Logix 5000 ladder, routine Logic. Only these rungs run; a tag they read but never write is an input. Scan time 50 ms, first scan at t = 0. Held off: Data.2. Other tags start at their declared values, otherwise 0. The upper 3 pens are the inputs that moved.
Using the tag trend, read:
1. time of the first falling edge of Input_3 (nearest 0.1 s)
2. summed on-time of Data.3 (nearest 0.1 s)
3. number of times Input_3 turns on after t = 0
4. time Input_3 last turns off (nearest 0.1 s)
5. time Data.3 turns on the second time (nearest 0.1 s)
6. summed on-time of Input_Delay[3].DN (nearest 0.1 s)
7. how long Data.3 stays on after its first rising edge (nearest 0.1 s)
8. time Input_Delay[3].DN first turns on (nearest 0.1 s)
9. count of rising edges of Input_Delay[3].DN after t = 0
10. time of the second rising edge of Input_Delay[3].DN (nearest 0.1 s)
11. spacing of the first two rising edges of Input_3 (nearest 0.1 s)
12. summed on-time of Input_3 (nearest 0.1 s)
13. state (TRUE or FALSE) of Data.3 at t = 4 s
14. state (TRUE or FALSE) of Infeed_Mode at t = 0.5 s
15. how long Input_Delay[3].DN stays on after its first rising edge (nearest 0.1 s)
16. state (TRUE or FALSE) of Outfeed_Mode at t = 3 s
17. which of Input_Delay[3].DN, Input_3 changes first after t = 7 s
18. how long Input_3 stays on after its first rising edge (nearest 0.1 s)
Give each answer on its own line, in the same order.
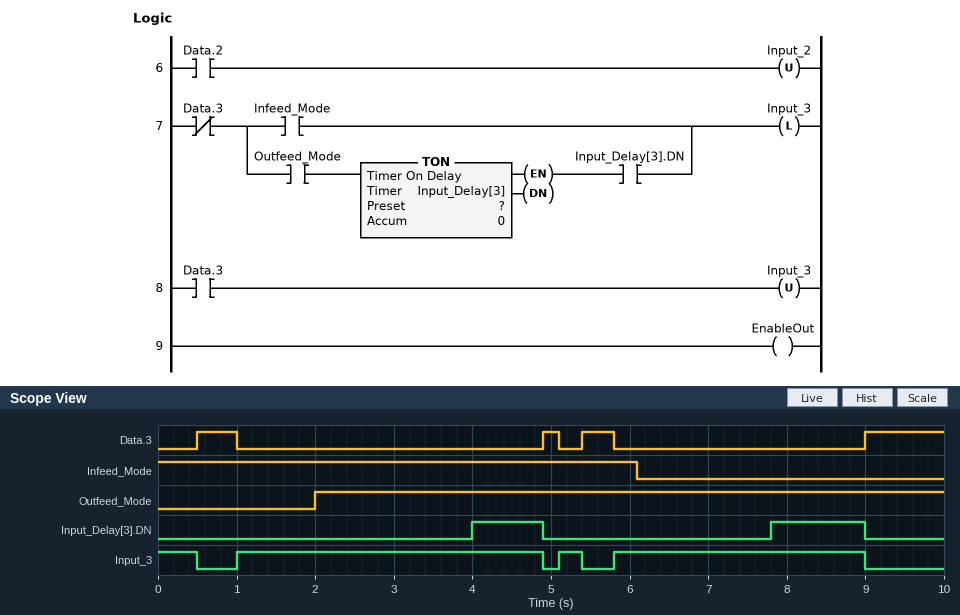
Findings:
0.5 s
2.1 s
3
9.0 s
4.9 s
2.1 s
0.5 s
4.0 s
2
7.8 s
4.1 s
7.9 s
FALSE
TRUE
0.9 s
TRUE
Input_Delay[3].DN
3.9 s
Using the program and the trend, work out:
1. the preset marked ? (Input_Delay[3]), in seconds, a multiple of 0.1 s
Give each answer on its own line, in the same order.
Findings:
2.0 s
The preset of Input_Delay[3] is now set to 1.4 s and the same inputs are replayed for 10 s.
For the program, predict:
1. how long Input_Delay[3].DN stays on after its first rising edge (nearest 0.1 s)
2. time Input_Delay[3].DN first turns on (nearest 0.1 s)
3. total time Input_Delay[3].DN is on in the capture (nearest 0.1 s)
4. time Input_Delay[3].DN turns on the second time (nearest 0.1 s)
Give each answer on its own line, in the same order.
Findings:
1.5 s
3.4 s
3.3 s
7.2 s
